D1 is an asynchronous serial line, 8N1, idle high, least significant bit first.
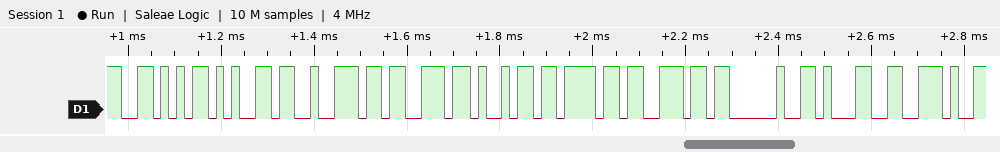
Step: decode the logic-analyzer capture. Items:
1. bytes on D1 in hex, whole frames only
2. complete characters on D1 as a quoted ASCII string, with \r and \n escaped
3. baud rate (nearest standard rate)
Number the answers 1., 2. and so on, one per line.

1. 56 65 72 73 69 6F 6E 20 31 2E
2. "Version 1."
3. 57600 baud
